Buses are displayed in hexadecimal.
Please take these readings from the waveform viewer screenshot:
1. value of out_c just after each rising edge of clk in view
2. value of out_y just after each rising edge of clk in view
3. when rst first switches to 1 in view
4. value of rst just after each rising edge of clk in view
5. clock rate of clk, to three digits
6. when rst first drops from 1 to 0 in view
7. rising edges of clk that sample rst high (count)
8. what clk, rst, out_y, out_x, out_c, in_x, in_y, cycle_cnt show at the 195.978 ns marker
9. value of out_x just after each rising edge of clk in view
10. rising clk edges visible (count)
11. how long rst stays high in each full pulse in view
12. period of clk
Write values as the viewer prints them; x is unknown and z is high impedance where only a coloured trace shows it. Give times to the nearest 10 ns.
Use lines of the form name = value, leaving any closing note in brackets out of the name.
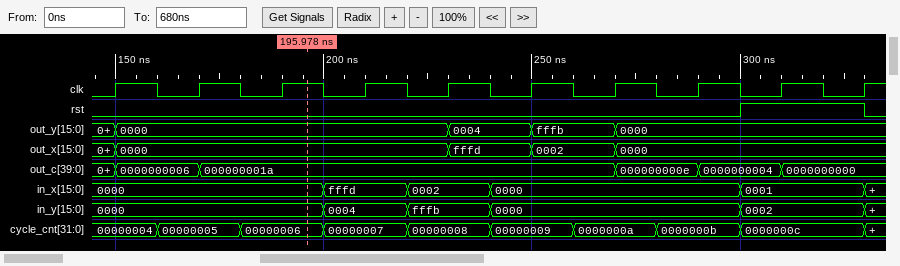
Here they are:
value of out_c just after each rising edge of clk in view = 0000000006, 000000001a, 000000001a, 000000001a, 000000001a, 000000001a, 000000000e, 0000000004, 0000000000, 0000000000
value of out_y just after each rising edge of clk in view = 0000, 0000, 0000, 0000, 0004, fffb, 0000, 0000, 0000, 0000
when rst first switches to 1 in view = 300 ns
value of rst just after each rising edge of clk in view = 0 0 0 0 0 0 0 0 1 0
clock rate of clk, to three digits = 50.0 MHz
when rst first drops from 1 to 0 in view = 330 ns
rising edges of clk that sample rst high = 2
what clk, rst, out_y, out_x, out_c, in_x, in_y, cycle_cnt show at the 195.978 ns marker = clk=1, rst=0, out_y=0000, out_x=0000, out_c=000000001a, in_x=0000, in_y=0000, cycle_cnt=00000006
value of out_x just after each rising edge of clk in view = 0000, 0000, 0000, 0000, fffd, 0002, 0000, 0000, 0000, 0000
rising clk edges visible = 10
how long rst stays high in each full pulse in view = 30 ns
period of clk = 20 ns
